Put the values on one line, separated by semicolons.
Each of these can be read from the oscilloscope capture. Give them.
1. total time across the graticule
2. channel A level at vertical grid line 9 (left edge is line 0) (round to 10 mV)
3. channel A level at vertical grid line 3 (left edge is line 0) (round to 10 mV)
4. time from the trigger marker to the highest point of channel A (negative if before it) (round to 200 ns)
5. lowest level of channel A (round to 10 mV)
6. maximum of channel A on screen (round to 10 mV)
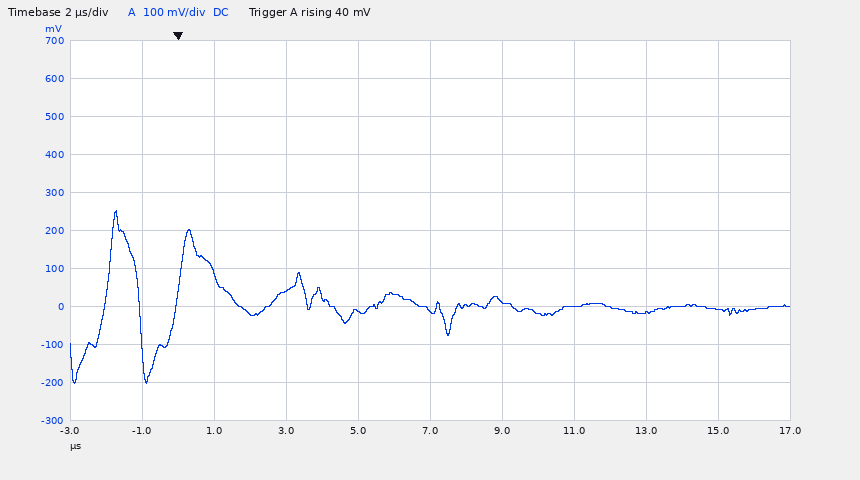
20 µs; -10 mV; 40 mV; -1.8 µs; -200 mV; 250 mV
